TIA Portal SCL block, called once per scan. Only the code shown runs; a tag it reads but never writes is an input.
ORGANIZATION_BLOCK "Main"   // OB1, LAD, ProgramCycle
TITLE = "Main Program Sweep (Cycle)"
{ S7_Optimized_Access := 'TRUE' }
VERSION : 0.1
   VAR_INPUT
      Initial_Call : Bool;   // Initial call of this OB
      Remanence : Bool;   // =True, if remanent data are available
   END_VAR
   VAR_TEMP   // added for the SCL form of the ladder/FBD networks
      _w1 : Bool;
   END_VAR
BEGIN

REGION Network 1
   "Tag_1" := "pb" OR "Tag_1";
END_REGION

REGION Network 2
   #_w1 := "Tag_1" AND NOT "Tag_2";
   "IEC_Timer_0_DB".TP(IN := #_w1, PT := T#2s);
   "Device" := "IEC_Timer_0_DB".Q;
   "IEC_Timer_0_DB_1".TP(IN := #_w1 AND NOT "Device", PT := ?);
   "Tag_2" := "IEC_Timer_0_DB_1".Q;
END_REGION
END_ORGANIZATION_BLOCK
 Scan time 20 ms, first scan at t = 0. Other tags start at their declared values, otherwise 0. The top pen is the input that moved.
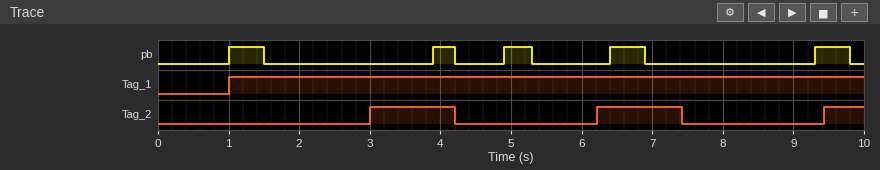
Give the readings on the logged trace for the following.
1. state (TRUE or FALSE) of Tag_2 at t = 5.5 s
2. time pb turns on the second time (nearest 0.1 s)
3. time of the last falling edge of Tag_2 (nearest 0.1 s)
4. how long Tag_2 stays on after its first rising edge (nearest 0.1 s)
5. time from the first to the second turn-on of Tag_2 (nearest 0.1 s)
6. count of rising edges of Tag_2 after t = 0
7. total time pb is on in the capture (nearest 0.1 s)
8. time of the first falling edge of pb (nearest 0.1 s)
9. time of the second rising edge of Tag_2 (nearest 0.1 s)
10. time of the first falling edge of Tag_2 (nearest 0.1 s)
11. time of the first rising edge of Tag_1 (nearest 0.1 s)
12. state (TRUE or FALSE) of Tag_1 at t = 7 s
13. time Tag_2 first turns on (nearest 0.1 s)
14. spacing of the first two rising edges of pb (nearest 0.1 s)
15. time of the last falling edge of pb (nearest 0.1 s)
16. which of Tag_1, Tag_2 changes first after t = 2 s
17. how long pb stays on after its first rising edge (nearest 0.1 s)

FALSE
3.9 s
7.4 s
1.2 s
3.2 s
3
2.2 s
1.5 s
6.2 s
4.2 s
1.0 s
TRUE
3.0 s
2.9 s
9.8 s
Tag_2
0.5 s
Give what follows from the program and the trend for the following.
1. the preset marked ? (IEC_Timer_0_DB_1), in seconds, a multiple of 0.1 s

1.2 s
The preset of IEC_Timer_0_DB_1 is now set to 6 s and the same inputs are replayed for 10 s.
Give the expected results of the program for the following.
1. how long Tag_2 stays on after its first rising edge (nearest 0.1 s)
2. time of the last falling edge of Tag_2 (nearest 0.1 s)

6.0 s
9.0 s
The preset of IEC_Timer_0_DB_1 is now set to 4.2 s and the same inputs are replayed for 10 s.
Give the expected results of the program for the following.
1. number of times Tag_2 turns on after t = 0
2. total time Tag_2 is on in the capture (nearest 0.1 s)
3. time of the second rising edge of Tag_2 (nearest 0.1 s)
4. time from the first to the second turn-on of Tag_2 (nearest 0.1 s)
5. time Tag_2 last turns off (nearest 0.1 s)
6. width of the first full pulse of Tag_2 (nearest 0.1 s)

2
5.0 s
9.2 s
6.2 s
7.2 s
4.2 s
